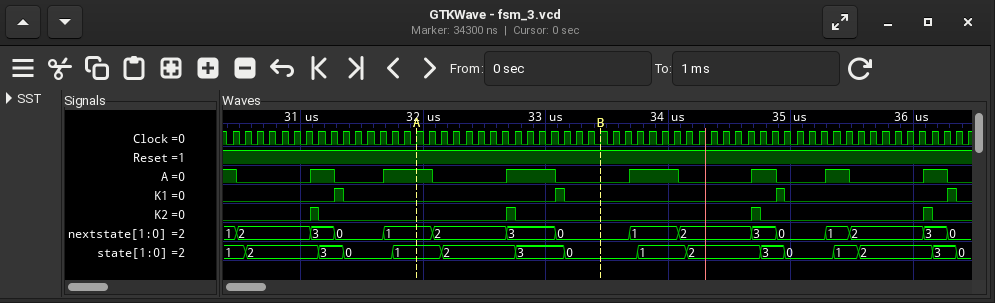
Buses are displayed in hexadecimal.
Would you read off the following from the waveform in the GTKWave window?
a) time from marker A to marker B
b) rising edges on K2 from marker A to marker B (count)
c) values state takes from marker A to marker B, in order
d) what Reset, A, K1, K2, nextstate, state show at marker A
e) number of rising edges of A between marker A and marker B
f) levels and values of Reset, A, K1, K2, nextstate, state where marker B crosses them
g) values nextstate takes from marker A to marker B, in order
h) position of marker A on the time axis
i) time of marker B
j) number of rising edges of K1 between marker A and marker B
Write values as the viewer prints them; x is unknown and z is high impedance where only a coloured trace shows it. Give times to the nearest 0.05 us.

1.5 us
1
1, 2, 3, 0
Reset=1, A=1, K1=0, K2=0, nextstate=1, state=1
1
Reset=1, A=0, K1=0, K2=0, nextstate=0, state=0
1, 2, 3, 0
31.95 us
33.45 us
1
